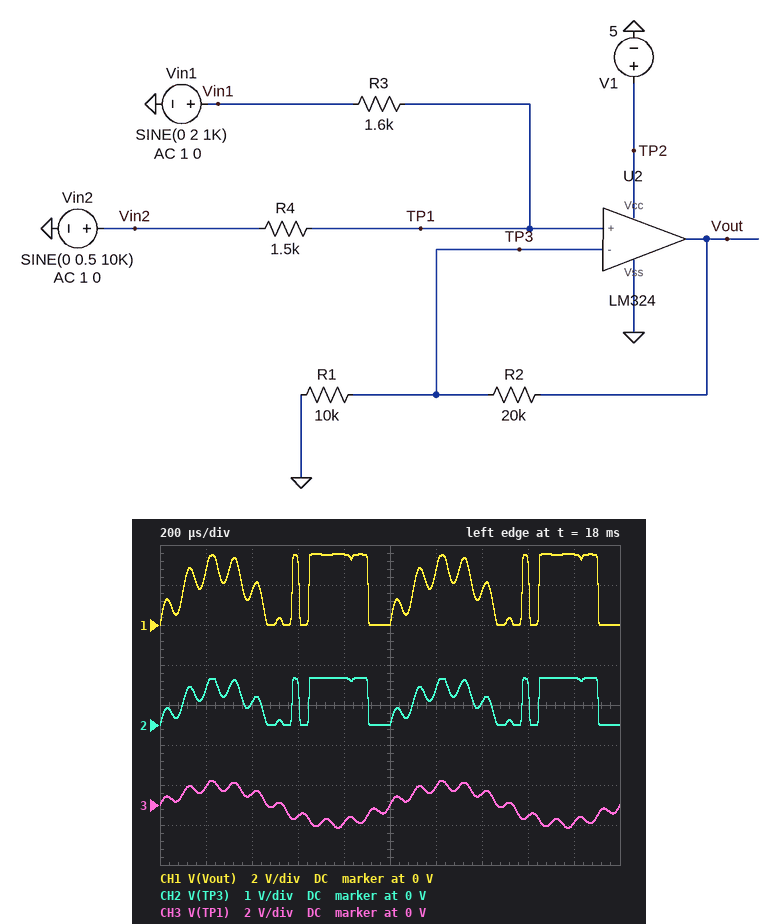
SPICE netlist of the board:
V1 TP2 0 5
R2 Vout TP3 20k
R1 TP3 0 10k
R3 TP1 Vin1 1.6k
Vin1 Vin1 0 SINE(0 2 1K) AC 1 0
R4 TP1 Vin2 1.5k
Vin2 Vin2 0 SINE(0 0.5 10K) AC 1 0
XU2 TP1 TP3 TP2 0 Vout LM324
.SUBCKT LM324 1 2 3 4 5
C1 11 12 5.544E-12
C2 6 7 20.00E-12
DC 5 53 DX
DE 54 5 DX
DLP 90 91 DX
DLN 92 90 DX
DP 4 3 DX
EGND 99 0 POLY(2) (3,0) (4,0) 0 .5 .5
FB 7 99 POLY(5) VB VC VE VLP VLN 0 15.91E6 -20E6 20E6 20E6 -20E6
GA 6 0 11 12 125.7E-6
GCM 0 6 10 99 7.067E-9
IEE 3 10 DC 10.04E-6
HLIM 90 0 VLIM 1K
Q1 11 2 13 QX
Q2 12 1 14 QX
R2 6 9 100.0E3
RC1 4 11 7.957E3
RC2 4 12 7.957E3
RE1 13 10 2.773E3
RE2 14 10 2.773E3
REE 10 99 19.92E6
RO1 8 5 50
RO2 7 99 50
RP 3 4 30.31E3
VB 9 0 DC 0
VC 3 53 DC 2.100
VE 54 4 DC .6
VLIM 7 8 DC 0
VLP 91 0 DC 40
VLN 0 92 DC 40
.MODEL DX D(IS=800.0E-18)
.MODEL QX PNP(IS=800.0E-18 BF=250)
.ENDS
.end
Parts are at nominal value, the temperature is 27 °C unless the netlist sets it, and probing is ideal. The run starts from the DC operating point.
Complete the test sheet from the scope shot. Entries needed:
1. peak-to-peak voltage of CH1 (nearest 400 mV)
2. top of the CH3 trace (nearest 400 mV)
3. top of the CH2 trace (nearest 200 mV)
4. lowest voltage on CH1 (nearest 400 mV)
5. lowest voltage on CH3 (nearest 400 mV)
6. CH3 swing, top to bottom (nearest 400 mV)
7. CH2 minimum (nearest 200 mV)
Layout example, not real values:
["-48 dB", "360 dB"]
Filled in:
["3.6 V", "1.2 V", "1.2 V", "0 V", "-1.2 V", "2.4 V", "0 V"]
